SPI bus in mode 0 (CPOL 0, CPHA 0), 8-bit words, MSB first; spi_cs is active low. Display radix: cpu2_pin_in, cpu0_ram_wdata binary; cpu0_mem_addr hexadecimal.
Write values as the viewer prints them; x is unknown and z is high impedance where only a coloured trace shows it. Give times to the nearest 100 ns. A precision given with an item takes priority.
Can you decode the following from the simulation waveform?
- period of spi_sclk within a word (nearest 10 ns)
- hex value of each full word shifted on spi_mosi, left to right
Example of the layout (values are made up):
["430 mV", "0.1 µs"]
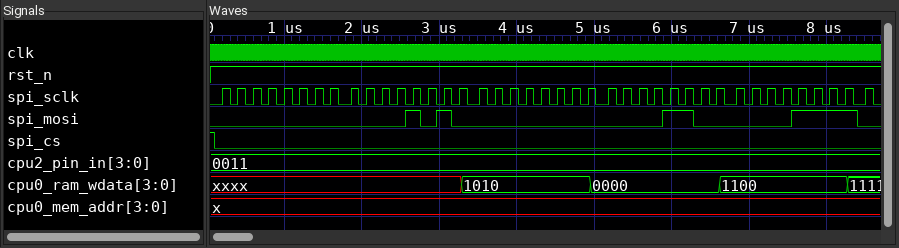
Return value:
["200 ns", "00, 0A, 00, 0C, 0F"]
